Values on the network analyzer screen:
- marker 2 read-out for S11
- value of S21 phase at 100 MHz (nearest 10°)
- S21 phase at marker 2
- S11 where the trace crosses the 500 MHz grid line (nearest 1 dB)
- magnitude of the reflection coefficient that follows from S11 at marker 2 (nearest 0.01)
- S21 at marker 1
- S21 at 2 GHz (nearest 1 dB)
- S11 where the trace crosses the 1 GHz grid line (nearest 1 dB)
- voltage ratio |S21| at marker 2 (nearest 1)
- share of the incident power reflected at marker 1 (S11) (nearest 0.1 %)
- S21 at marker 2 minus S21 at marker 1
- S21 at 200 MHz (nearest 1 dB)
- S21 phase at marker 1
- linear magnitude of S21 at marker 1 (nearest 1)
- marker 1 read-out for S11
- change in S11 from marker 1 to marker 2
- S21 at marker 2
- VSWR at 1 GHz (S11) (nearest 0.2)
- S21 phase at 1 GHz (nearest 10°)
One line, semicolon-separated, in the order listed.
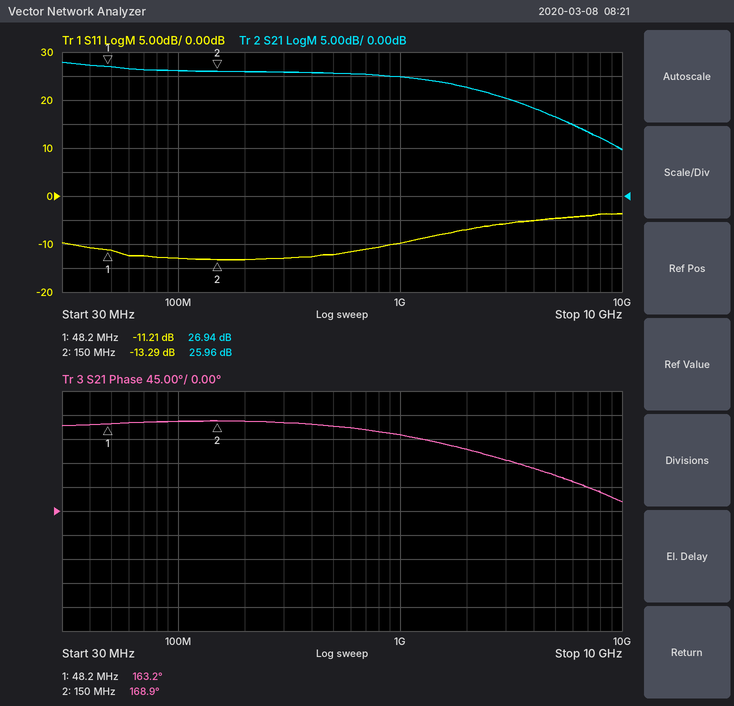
-13.29 dB; 170°; 168.9°; -12 dB; 0.22; 26.94 dB; 23 dB; -10 dB; 20; 7.6 %; -0.98 dB; 26 dB; 163.2°; 22; -11.21 dB; -2.08 dB; 25.96 dB; 2.0; 140°
